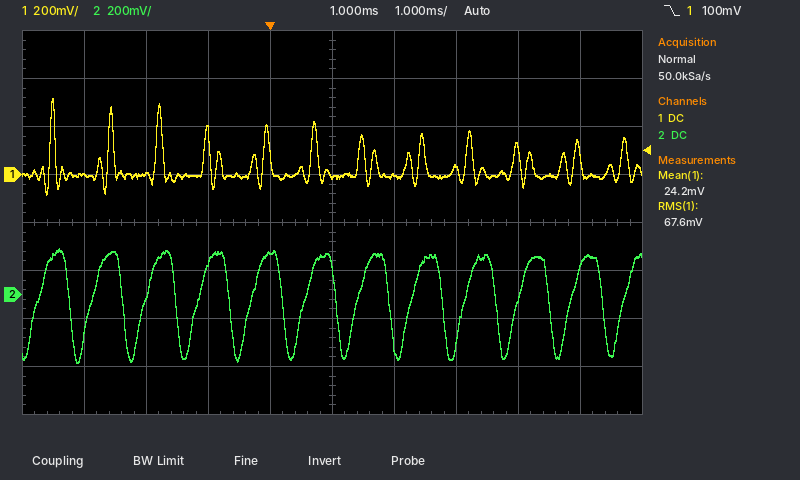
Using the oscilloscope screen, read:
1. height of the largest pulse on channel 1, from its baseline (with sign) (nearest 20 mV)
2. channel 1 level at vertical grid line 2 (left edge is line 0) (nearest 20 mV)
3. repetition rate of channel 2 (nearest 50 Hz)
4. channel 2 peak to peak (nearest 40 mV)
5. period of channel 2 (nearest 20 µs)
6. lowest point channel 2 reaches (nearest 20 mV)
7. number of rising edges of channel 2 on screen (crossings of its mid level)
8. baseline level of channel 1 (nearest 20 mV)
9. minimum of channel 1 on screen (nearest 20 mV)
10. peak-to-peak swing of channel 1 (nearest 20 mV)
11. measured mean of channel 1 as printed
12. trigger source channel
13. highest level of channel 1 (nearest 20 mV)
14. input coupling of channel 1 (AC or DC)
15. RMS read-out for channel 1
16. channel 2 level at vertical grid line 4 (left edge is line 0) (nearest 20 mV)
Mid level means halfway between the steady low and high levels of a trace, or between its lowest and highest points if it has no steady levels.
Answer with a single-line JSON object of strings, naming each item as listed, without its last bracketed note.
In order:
{"height of the largest pulse on channel 1, from its baseline (with sign)": "+320 mV", "channel 1 level at vertical grid line 2 (left edge is line 0)": "0 mV", "repetition rate of channel 2": "1.15 kHz", "channel 2 peak to peak": "480 mV", "period of channel 2": "860 µs", "lowest point channel 2 reaches": "-280 mV", "number of rising edges of channel 2 on screen": "12", "baseline level of channel 1": "0 mV", "minimum of channel 1 on screen": "-80 mV", "peak-to-peak swing of channel 1": "400 mV", "measured mean of channel 1 as printed": "24.2 mV", "trigger source channel": "channel 1", "highest level of channel 1": "320 mV", "input coupling of channel 1": "DC", "RMS read-out for channel 1": "67.6 mV", "channel 2 level at vertical grid line 4 (left edge is line 0)": "180 mV"}
